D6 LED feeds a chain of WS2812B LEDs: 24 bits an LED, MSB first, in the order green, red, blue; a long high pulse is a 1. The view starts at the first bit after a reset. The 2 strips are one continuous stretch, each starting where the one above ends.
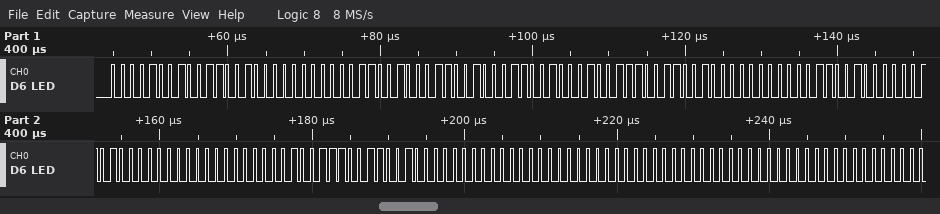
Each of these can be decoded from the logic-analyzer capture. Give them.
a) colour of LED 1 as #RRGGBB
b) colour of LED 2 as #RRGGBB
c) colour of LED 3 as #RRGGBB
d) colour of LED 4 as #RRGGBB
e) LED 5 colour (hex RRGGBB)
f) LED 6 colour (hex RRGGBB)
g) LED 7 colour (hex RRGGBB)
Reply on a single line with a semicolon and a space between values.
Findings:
#320900; #323232; #322700; #053200; #270032; #000000; #000000
